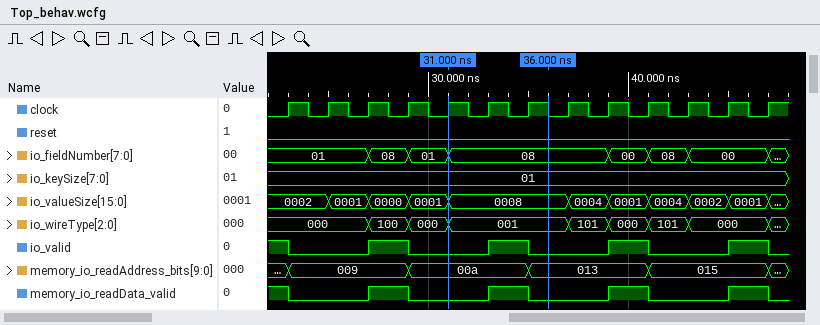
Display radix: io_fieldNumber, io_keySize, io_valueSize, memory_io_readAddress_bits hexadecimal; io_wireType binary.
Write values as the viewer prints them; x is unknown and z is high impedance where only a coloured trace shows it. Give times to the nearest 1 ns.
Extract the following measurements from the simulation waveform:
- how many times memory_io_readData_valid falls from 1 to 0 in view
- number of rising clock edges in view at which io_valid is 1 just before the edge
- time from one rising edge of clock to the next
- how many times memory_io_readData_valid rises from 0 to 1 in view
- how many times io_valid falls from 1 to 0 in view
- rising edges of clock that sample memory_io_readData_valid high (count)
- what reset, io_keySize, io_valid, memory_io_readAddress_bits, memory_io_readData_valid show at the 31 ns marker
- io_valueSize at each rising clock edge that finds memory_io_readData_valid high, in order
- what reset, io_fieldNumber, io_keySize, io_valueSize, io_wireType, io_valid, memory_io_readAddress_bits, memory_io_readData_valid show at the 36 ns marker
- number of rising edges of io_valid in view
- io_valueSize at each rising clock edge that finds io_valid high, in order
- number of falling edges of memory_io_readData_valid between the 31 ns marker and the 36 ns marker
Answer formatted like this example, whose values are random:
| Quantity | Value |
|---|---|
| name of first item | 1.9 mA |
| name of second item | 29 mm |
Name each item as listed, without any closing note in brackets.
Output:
| Quantity | Value |
|---|---|
| how many times memory_io_readData_valid falls from 1 to 0 in view | 5 |
| number of rising clock edges in view at which io_valid is 1 just before the edge | 5 |
| time from one rising edge of clock to the next | 2 ns |
| how many times memory_io_readData_valid rises from 0 to 1 in view | 4 |
| how many times io_valid falls from 1 to 0 in view | 5 |
| rising edges of clock that sample memory_io_readData_valid high | 5 |
| what reset, io_keySize, io_valid, memory_io_readAddress_bits, memory_io_readData_valid show at the 31 ns marker | reset=0, io_keySize=01, io_valid=0, memory_io_readAddress_bits=00a, memory_io_readData_valid=0 |
| io_valueSize at each rising clock edge that finds memory_io_readData_valid high, in order | 0002, 0000, 0008, 0001, 0001 |
| what reset, io_fieldNumber, io_keySize, io_valueSize, io_wireType, io_valid, memory_io_readAddress_bits, memory_io_readData_valid show at the 36 ns marker | reset=0, io_fieldNumber=08, io_keySize=01, io_valueSize=0008, io_wireType=001, io_valid=0, memory_io_readAddress_bits=013, memory_io_readData_valid=0 |
| number of rising edges of io_valid in view | 4 |
| io_valueSize at each rising clock edge that finds io_valid high, in order | 0002, 0000, 0008, 0001, 0001 |
| number of falling edges of memory_io_readData_valid between the 31 ns marker and the 36 ns marker | 1 |
